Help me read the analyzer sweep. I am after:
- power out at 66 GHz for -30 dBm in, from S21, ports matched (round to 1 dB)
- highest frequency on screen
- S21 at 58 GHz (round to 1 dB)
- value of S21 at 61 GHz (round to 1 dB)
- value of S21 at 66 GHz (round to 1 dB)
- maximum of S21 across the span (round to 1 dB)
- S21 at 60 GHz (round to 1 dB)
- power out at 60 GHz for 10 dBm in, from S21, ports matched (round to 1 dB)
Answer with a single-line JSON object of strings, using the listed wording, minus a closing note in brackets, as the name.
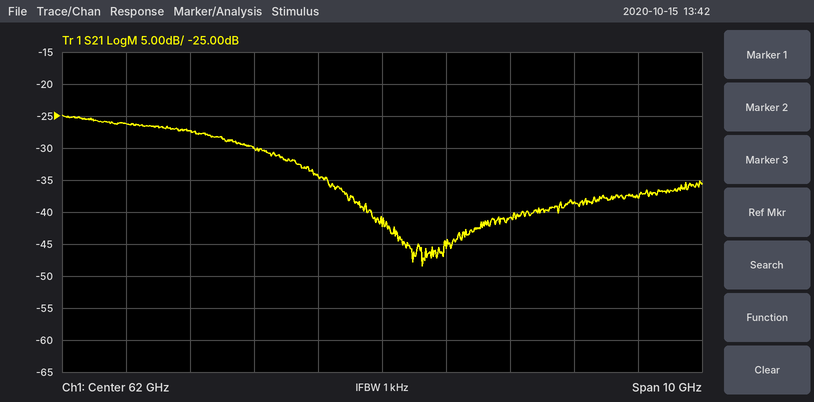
{"power out at 66 GHz for -30 dBm in, from S21, ports matched": "-68 dBm", "highest frequency on screen": "67 GHz", "S21 at 58 GHz": "-26 dB", "value of S21 at 61 GHz": "-34 dB", "value of S21 at 66 GHz": "-38 dB", "maximum of S21 across the span": "-25 dB", "S21 at 60 GHz": "-30 dB", "power out at 60 GHz for 10 dBm in, from S21, ports matched": "-20 dBm"}
